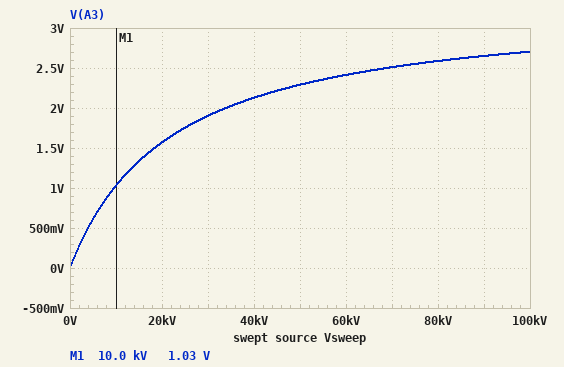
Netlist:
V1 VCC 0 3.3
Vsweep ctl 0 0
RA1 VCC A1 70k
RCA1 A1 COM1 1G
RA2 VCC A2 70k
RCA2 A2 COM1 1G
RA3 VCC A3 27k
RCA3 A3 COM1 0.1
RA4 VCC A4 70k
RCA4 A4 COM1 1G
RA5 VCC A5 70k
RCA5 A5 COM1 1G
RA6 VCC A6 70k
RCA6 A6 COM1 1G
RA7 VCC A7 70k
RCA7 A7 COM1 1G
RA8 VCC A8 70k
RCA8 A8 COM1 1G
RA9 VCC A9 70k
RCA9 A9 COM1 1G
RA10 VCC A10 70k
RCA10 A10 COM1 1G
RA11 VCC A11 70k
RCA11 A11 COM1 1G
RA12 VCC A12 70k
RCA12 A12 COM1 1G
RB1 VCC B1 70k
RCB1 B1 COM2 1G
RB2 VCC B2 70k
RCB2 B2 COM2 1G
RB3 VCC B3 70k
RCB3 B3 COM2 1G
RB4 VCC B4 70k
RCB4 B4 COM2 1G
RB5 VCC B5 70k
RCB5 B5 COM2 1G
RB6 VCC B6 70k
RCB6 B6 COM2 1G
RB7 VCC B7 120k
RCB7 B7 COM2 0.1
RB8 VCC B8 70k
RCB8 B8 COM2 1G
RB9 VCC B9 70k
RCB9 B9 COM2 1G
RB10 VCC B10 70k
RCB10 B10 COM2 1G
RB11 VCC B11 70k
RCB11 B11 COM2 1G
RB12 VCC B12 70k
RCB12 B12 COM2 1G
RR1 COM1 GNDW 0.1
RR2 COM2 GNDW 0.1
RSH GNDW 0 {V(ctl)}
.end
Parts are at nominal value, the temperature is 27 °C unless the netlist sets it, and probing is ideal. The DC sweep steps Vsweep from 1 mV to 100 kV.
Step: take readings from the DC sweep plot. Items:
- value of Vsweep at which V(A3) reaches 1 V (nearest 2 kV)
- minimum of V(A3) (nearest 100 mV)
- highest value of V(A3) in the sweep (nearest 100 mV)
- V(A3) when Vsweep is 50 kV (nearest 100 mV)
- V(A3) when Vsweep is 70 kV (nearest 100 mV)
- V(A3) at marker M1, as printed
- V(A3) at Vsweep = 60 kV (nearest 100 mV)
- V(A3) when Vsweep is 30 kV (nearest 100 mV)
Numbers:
10 kV
0 V
2.7 V
2.3 V
2.5 V
1.03 V
2.4 V
1.9 V
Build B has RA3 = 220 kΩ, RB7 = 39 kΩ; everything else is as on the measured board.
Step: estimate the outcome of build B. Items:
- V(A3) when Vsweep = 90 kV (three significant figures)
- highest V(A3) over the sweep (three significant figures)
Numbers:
2.41 V
2.48 V
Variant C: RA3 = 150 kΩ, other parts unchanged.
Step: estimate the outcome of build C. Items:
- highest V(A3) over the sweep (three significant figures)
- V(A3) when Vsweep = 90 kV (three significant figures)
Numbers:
1.98 V
1.90 V
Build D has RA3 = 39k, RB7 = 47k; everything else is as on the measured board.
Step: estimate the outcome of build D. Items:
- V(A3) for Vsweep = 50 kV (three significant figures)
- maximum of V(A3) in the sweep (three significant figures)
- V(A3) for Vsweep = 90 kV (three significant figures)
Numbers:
2.31 V
2.72 V
2.67 V
